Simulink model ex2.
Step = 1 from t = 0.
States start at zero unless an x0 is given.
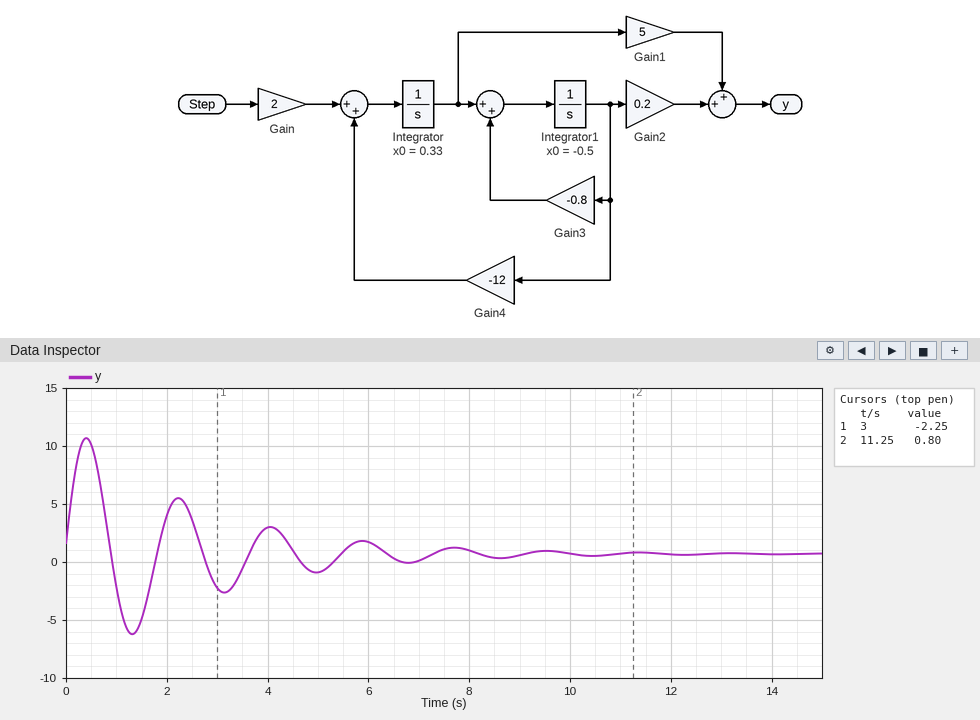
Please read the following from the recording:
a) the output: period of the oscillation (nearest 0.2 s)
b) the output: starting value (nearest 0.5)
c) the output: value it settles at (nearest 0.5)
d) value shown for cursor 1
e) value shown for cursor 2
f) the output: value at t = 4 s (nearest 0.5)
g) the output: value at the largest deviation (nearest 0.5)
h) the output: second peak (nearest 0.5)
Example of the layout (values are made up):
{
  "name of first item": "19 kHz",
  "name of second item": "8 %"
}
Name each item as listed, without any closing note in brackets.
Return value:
{
  "the output: period of the oscillation": "1.8 s",
  "the output: starting value": "1.5",
  "the output: value it settles at": "0.5",
  "value shown for cursor 1": "-2.25",
  "value shown for cursor 2": "0.80",
  "the output: value at t = 4 s": "3.0",
  "the output: value at the largest deviation": "10.5",
  "the output: second peak": "5.5"
}
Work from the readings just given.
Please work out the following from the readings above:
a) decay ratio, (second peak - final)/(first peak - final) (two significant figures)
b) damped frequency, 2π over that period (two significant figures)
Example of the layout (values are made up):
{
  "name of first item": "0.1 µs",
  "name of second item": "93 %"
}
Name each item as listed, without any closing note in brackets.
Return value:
{
  "decay ratio, (second peak - final)/(first peak - final)": "0.50",
  "damped frequency, 2π over that period": "3.5 rad/s"
}
